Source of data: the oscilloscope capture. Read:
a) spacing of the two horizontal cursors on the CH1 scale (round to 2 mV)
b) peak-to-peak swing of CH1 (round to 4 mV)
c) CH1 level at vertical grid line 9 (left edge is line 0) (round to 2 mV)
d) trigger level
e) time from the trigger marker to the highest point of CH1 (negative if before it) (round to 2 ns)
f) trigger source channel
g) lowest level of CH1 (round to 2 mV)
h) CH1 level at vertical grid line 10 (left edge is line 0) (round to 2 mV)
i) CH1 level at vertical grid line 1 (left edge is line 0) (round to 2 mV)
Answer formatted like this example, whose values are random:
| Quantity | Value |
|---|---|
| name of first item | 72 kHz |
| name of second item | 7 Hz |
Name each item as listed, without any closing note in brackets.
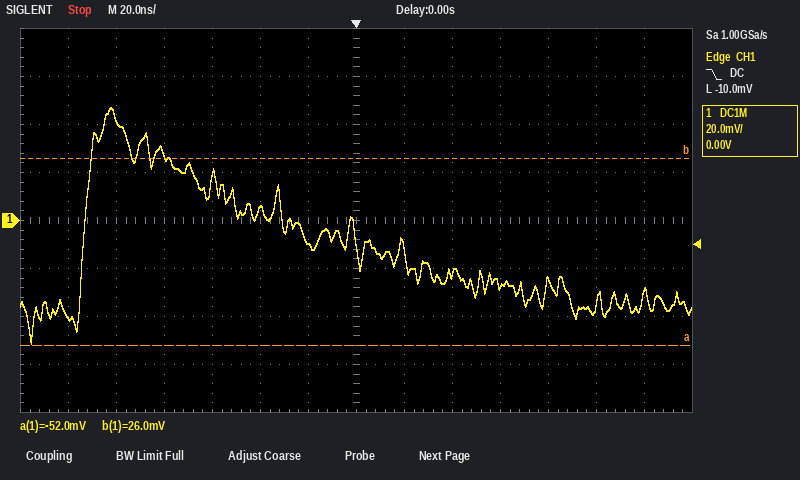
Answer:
| Quantity | Value |
|---|---|
| spacing of the two horizontal cursors on the CH1 scale | 78 mV |
| peak-to-peak swing of CH1 | 100 mV |
| CH1 level at vertical grid line 9 (left edge is line 0) | -22 mV |
| trigger level | -10.0 mV |
| time from the trigger marker to the highest point of CH1 (negative if before it) | -102 ns |
| trigger source channel | CH1 |
| lowest level of CH1 | -52 mV |
| CH1 level at vertical grid line 10 (left edge is line 0) | -28 mV |
| CH1 level at vertical grid line 1 (left edge is line 0) | -40 mV |
